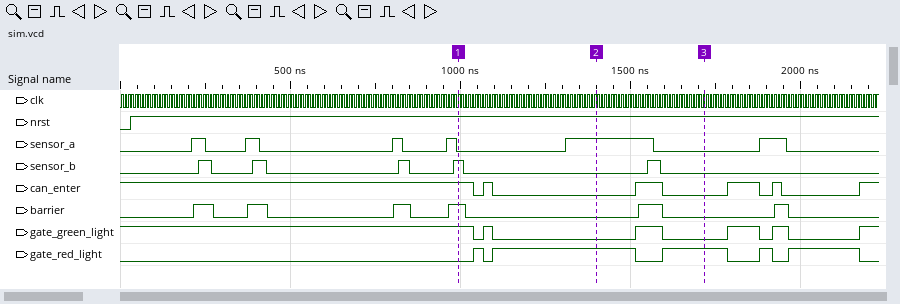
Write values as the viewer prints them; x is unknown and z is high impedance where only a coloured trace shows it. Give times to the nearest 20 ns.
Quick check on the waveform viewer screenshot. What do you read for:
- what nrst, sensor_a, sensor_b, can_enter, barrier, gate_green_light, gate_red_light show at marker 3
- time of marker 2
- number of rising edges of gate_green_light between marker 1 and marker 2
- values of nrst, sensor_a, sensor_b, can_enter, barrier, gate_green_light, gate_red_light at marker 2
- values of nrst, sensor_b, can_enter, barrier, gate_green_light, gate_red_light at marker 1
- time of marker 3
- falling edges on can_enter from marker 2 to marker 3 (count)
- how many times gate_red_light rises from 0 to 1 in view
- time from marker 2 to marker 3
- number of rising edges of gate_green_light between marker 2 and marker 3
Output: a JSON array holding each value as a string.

["nrst=1, sensor_a=0, sensor_b=0, can_enter=0, barrier=0, gate_green_light=0, gate_red_light=1", "1400 ns", "1", "nrst=1, sensor_a=1, sensor_b=0, can_enter=0, barrier=0, gate_green_light=0, gate_red_light=1", "nrst=1, sensor_b=1, can_enter=1, barrier=1, gate_green_light=1, gate_red_light=0", "1720 ns", "1", "5", "320 ns", "1"]
